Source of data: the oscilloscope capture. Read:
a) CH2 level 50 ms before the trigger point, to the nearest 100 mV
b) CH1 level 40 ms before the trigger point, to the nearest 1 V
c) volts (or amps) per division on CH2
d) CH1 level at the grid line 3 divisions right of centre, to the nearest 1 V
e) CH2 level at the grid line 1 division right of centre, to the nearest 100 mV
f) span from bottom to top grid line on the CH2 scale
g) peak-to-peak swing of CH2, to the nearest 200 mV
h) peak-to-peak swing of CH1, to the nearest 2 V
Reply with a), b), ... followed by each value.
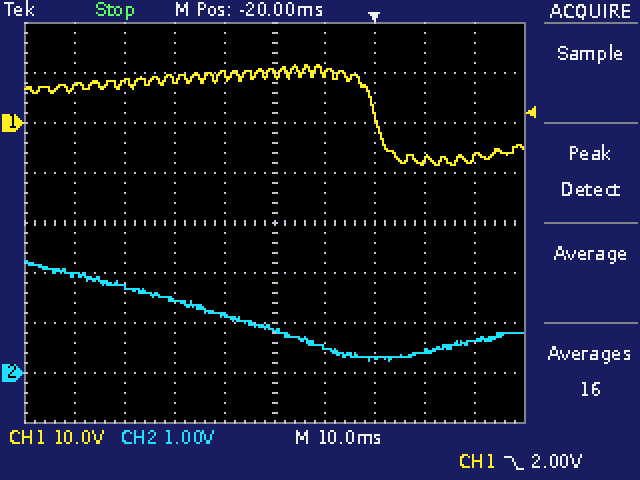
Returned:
a) 1.7 V
b) 9 V
c) 1 V
d) -7 V
e) 500 mV
f) 8 V
g) 2.0 V
h) 20 V
